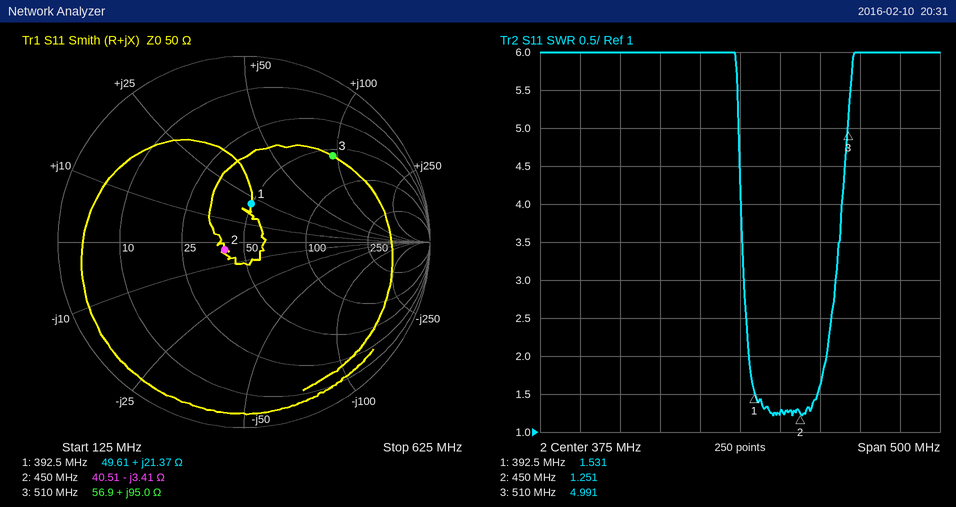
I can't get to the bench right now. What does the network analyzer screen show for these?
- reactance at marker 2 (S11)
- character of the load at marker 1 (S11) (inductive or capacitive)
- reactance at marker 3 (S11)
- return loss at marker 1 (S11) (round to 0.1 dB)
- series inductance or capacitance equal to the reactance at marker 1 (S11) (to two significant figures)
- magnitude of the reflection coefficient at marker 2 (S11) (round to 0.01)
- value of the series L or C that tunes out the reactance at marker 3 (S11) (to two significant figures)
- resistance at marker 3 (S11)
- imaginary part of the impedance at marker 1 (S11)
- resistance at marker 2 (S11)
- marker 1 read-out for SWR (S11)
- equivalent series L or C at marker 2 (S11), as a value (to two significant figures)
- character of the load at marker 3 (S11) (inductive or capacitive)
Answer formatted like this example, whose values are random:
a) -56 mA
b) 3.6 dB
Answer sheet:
a) -3.41 Ω
b) inductive
c) +95.0 Ω
d) 13.6 dB
e) 8.7 nH
f) 0.11
g) 3.3 pF
h) 56.9 Ω
i) +21.37 Ω
j) 40.51 Ω
k) 1.531
l) 100 pF
m) inductive
